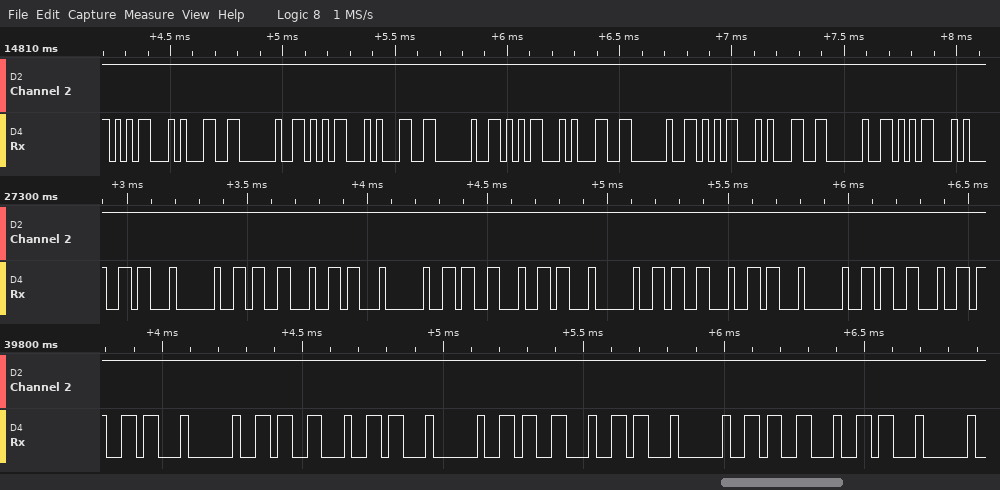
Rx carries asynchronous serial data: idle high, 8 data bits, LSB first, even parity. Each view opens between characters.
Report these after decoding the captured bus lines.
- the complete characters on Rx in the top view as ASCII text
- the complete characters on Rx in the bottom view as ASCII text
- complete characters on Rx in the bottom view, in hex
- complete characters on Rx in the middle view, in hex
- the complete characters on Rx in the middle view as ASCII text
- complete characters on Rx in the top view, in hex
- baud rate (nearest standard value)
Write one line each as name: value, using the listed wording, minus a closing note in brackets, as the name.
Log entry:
the complete characters on Rx in the top view as ASCII text: "51 51 51 51 5"
the complete characters on Rx in the bottom view as ASCII text: "6 36 36 36"
complete characters on Rx in the bottom view, in hex: 36, 20, 33, 36, 20, 33, 36, 20, 33, 36
complete characters on Rx in the middle view, in hex: 36, 20, 33, 36, 20, 33, 36, 20, 33, 36, 20, 33
the complete characters on Rx in the middle view as ASCII text: "6 36 36 36 3"
complete characters on Rx in the top view, in hex: 35, 31, 20, 35, 31, 20, 35, 31, 20, 35, 31, 20, 35
baud rate: 38400 baud
